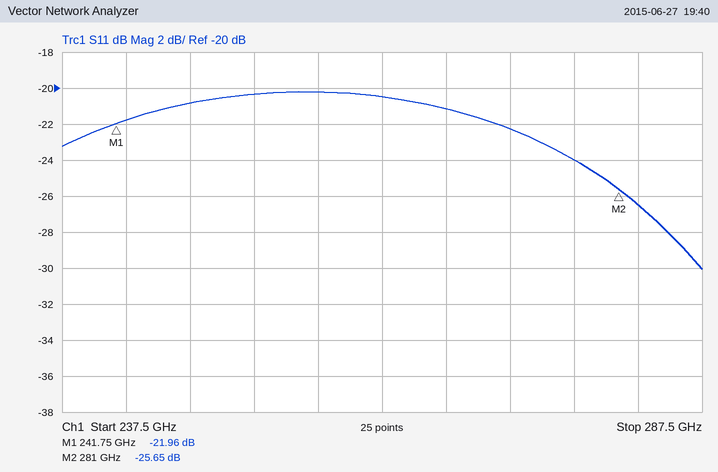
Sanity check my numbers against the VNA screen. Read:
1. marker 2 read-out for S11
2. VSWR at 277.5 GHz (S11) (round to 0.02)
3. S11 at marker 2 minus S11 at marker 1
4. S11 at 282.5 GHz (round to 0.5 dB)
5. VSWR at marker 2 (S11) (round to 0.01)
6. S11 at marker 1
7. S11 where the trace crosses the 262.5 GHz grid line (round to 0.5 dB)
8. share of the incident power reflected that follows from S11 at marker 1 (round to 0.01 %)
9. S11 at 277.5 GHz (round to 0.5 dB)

-25.65 dB
1.14
-3.69 dB
-26.5 dB
1.11
-21.96 dB
-20.5 dB
0.64 %
-24.0 dB
